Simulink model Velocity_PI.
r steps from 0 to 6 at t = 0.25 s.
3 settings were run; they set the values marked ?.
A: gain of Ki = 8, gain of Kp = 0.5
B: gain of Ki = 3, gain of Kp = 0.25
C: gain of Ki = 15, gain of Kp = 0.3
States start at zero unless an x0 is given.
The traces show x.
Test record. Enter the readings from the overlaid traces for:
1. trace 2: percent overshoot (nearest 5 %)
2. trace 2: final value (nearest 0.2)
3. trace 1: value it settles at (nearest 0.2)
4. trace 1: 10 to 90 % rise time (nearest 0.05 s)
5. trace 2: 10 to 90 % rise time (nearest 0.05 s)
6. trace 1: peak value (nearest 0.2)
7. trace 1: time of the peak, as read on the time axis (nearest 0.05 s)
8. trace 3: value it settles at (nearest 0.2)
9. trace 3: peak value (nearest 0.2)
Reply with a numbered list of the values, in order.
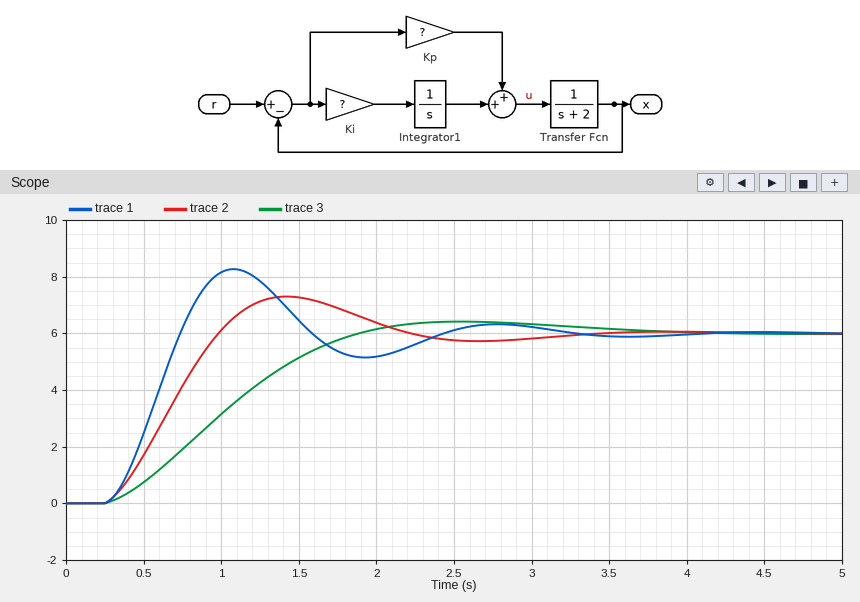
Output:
1. 20 %
2. 6.0
3. 6.0
4. 0.35 s
5. 0.55 s
6. 8.2
7. 1.10 s
8. 6.0
9. 6.4
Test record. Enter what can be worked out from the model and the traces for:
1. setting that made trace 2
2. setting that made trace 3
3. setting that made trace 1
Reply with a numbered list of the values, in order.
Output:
1. A
2. B
3. C
